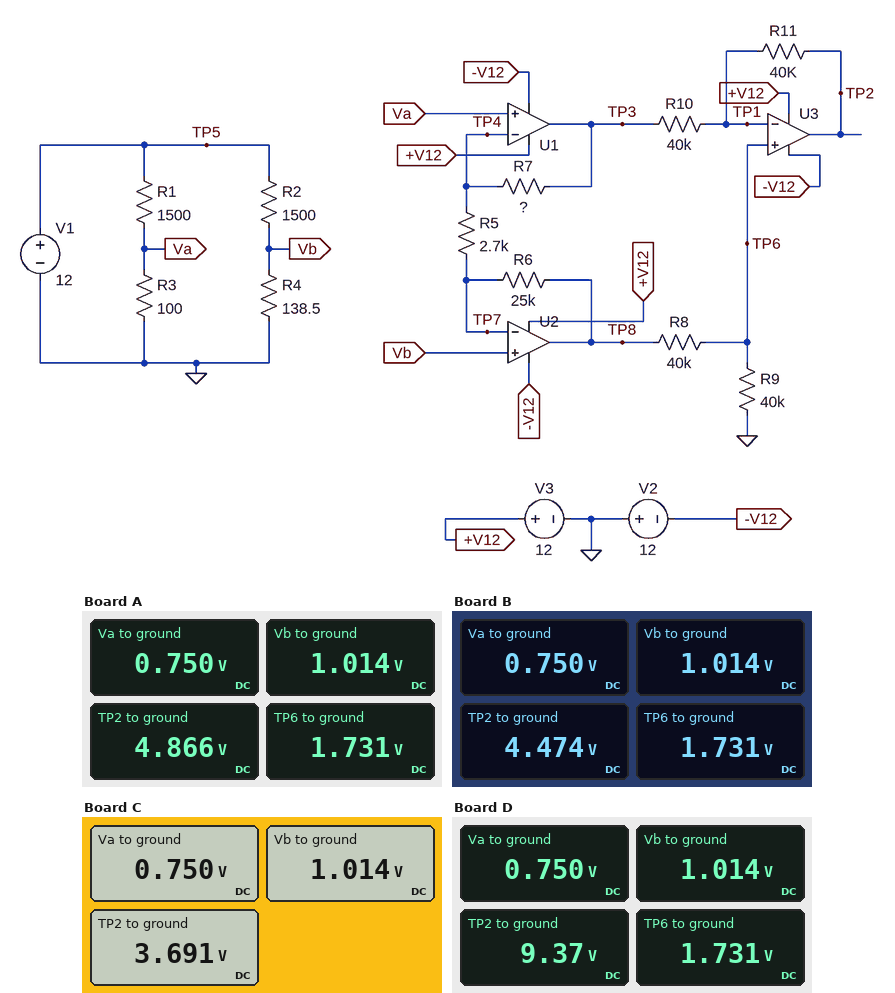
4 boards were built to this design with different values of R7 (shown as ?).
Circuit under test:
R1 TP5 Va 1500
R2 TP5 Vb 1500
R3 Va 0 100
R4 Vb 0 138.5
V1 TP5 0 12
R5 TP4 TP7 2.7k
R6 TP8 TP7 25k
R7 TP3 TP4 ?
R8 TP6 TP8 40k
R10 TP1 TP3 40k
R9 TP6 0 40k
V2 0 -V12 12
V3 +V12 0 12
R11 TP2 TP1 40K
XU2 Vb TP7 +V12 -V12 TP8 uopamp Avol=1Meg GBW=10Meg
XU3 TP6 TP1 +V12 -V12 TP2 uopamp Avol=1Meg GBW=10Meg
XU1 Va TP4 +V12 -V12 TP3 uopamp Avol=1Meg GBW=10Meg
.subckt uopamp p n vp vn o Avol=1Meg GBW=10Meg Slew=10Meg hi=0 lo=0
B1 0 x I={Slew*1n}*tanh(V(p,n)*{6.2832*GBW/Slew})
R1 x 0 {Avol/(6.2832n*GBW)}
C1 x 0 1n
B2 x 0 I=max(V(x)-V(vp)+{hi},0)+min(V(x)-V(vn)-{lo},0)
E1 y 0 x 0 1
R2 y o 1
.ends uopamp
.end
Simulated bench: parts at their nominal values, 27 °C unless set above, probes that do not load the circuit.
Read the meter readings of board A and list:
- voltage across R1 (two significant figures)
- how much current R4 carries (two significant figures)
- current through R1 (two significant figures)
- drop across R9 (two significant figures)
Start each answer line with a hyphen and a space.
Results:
- 11 V
- 7.3 mA
- 7.5 mA
- 1.7 V
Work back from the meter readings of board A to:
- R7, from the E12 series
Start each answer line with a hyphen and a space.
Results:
- 22 kΩ
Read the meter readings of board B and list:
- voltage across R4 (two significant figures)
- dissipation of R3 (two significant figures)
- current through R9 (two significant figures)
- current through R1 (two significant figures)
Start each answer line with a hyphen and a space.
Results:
- 1.0 V
- 5.6 mW
- 43 µA
- 7.5 mA
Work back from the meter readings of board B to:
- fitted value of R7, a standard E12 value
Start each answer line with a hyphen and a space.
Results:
- 18 kΩ
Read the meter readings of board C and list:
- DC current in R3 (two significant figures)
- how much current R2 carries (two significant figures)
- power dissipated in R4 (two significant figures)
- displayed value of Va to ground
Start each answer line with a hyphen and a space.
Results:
- 7.5 mA
- 7.3 mA
- 7.4 mW
- 0.750 V
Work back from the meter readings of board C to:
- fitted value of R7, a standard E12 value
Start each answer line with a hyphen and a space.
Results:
- 10 kΩ
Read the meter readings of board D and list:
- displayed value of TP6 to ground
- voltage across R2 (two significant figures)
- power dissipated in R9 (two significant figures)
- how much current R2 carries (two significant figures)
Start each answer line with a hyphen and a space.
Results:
- 1.731 V
- 11 V
- 75 µW
- 7.3 mA
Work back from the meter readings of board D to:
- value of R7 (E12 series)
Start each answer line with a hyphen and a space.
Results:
- 68 kΩ
